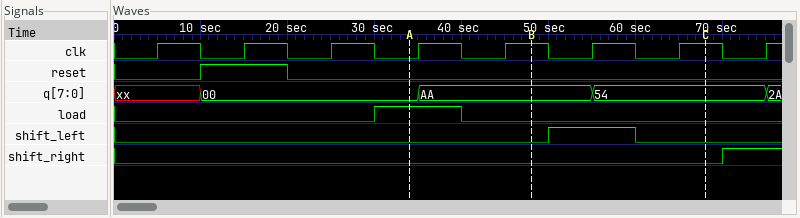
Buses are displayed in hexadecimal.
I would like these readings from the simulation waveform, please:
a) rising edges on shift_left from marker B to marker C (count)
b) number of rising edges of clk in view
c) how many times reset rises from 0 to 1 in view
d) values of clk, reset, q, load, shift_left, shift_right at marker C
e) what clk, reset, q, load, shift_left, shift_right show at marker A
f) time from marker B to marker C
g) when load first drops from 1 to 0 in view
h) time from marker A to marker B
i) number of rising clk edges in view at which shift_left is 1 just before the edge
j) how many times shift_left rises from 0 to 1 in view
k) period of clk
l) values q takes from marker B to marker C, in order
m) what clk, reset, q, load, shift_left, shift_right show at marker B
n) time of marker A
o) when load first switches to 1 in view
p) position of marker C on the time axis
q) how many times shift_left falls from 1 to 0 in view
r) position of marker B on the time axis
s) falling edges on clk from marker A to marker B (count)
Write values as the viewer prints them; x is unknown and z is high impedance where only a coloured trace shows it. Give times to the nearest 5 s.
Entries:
1
8
1
clk=1, reset=0, q=54, load=0, shift_left=0, shift_right=0
clk=0, reset=0, q=00, load=1, shift_left=0, shift_right=0
20 s
40 s
15 s
1
1
10 s
AA, 54
clk=1, reset=0, q=AA, load=0, shift_left=0, shift_right=0
35 s
30 s
70 s
1
50 s
1
